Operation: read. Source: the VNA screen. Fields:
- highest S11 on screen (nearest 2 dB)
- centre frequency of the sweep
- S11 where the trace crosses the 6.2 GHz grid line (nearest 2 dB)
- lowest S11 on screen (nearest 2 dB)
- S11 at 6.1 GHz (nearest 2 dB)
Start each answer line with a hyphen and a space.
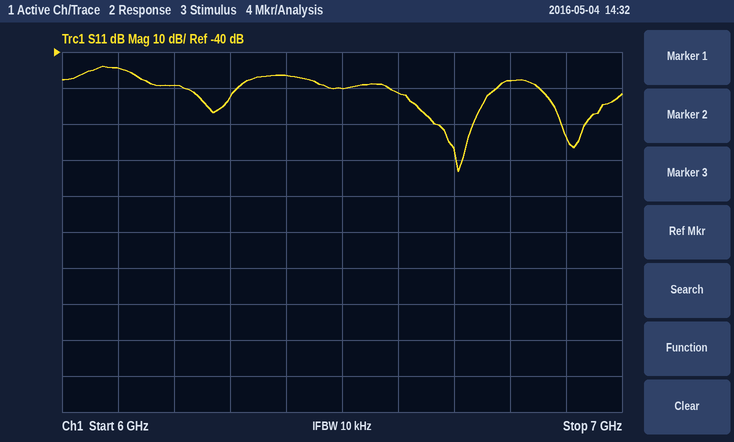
- -44 dB
- 6.5 GHz
- -50 dB
- -74 dB
- -44 dB
